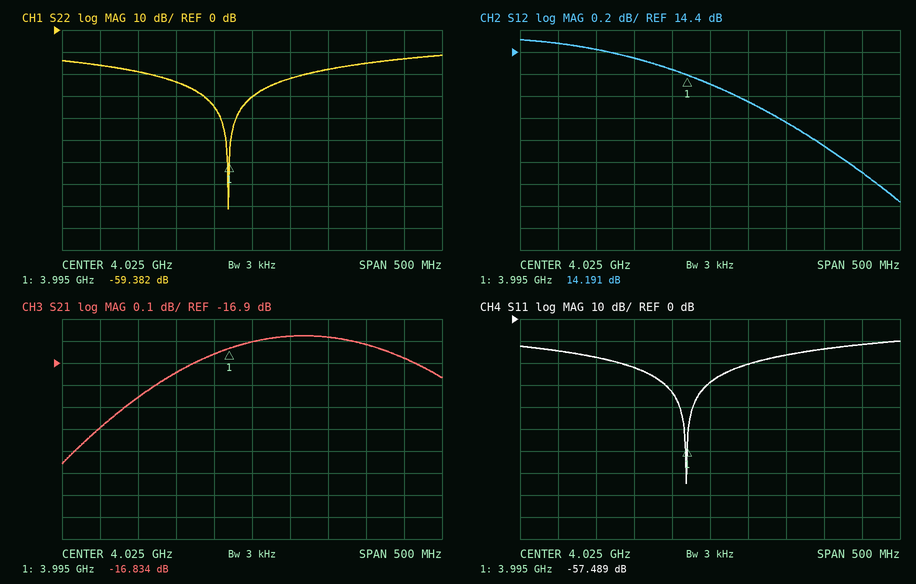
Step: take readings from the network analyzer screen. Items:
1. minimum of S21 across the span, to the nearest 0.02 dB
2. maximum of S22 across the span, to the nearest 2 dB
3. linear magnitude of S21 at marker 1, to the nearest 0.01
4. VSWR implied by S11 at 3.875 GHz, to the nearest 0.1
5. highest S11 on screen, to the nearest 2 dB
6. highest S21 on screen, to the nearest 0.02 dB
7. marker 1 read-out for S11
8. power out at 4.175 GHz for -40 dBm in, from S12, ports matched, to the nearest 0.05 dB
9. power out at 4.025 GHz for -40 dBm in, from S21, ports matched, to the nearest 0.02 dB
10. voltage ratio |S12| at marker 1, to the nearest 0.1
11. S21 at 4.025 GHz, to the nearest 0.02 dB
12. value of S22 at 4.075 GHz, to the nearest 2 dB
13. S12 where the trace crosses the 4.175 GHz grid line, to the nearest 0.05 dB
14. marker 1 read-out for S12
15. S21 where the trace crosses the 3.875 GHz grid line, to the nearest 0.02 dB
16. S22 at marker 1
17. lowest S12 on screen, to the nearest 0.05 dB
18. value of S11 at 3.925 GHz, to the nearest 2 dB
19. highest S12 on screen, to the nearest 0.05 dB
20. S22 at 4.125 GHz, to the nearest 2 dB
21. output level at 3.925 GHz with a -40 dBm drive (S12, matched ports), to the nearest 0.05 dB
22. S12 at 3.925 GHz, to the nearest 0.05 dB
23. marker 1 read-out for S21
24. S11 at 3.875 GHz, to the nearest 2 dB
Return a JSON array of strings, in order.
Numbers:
["-17.36 dB", "-12 dB", "0.14", "1.3", "-10 dB", "-16.78 dB", "-57.489 dB", "-26.45 dBm", "-56.80 dBm", "5.1", "-16.80 dB", "-22 dB", "13.55 dB", "14.191 dB", "-17.06 dB", "-59.382 dB", "13.05 dB", "-22 dB", "14.50 dB", "-18 dB", "-25.65 dBm", "14.35 dB", "-16.834 dB", "-18 dB"]
